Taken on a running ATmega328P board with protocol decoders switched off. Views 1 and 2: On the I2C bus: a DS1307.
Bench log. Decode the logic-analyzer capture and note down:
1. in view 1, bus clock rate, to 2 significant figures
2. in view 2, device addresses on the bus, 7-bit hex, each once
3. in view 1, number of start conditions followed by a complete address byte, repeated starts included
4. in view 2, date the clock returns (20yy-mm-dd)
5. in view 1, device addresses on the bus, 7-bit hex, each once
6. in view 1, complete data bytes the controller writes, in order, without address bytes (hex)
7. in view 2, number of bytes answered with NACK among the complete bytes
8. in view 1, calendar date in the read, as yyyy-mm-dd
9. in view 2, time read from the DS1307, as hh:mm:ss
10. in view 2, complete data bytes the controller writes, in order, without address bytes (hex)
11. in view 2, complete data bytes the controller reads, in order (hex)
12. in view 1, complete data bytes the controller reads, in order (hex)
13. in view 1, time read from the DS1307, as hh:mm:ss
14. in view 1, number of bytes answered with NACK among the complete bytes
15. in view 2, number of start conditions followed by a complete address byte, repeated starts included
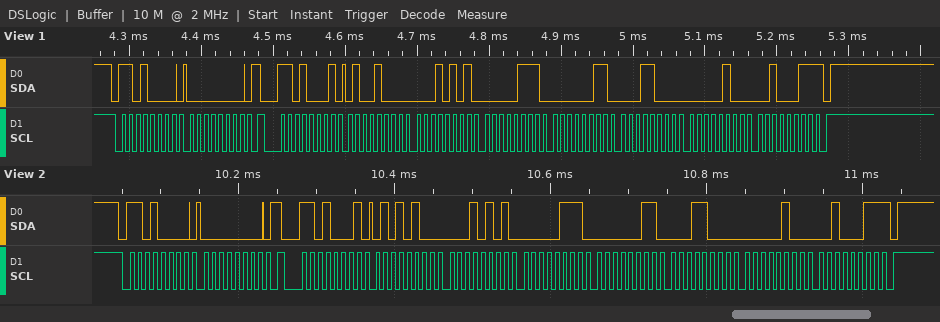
100 kHz
0x68
2
2023-04-18
0x68
00
1
2023-04-18
07:15:54
00
54 15 07 03 18 04 23
48 15 07 03 18 04 23
07:15:48
1
2
